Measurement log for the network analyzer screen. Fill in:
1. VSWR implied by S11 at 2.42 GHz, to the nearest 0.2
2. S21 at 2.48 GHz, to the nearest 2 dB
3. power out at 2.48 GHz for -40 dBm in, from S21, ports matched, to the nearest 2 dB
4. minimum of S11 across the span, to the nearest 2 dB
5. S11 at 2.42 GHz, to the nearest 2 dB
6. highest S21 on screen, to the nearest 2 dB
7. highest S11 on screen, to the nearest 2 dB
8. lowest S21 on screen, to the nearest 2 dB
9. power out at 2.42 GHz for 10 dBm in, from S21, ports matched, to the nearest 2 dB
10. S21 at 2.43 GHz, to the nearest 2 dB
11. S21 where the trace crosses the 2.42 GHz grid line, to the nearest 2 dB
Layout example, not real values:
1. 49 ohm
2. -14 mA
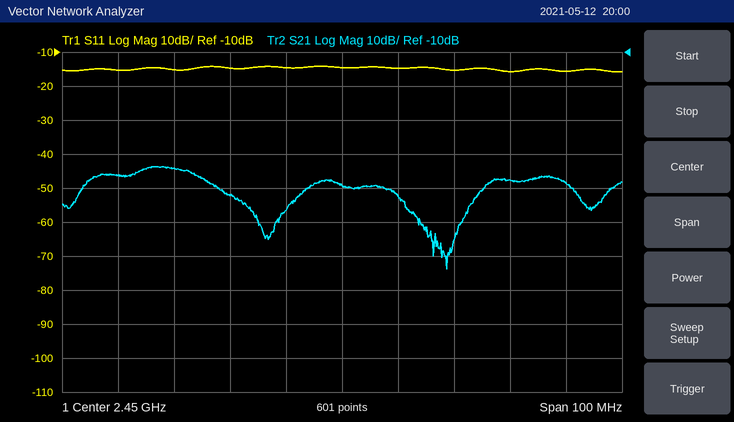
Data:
1. 1.4
2. -48 dB
3. -88 dBm
4. -16 dB
5. -16 dB
6. -44 dB
7. -14 dB
8. -74 dB
9. -34 dBm
10. -52 dB
11. -44 dB
